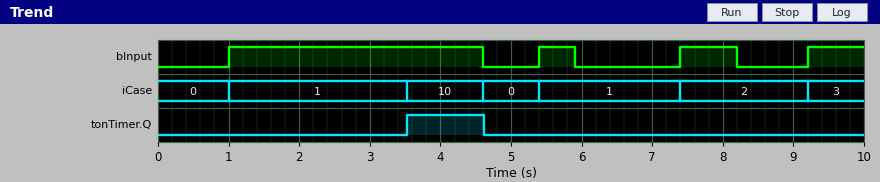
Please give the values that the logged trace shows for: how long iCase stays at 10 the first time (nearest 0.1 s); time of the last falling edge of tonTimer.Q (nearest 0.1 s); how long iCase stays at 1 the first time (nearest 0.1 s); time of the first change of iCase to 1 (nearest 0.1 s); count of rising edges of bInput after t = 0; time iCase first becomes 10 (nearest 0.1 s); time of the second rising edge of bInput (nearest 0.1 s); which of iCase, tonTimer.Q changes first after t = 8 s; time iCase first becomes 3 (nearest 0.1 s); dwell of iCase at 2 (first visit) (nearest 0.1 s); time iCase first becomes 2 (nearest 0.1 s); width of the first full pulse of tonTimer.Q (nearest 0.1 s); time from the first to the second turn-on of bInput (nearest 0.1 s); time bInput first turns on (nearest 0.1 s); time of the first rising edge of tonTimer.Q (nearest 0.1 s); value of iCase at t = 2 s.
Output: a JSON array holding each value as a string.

["1.1 s", "4.6 s", "2.5 s", "1.0 s", "4", "3.5 s", "5.4 s", "iCase", "9.2 s", "1.8 s", "7.4 s", "1.1 s", "4.4 s", "1.0 s", "3.5 s", "1"]
